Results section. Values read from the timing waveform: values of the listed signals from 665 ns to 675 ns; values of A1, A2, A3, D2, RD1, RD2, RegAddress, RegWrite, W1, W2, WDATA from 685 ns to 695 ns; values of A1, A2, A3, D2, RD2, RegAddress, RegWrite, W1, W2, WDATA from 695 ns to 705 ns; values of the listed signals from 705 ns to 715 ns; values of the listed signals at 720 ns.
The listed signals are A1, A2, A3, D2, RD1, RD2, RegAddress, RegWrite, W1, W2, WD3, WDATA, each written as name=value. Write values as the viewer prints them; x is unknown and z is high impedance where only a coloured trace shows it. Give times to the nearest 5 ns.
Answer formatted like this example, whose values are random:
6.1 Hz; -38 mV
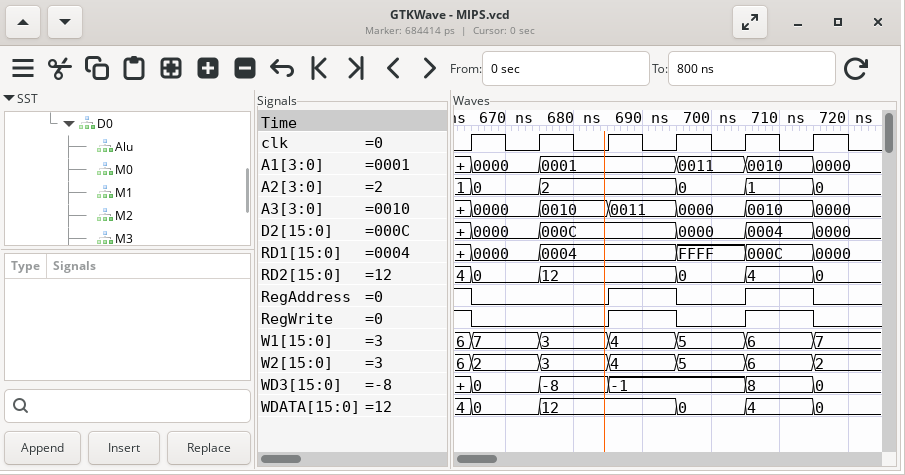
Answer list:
A1=0000, A2=0, A3=0000, D2=0000, RD1=0000, RD2=0, RegAddress=0, RegWrite=0, W1=7, W2=2, WD3=0, WDATA=0; A1=0001, A2=2, A3=0011, D2=000C, RD1=0004, RD2=12, RegAddress=1, RegWrite=1, W1=4, W2=4, WDATA=12; A1=0011, A2=0, A3=0000, D2=0000, RD2=0, RegAddress=0, RegWrite=0, W1=5, W2=5, WDATA=0; A1=0010, A2=1, A3=0010, D2=0004, RD1=000C, RD2=4, RegAddress=1, RegWrite=1, W1=6, W2=6, WD3=8, WDATA=4; A1=0000, A2=0, A3=0000, D2=0000, RD1=0000, RD2=0, RegAddress=0, RegWrite=0, W1=7, W2=2, WD3=0, WDATA=0
